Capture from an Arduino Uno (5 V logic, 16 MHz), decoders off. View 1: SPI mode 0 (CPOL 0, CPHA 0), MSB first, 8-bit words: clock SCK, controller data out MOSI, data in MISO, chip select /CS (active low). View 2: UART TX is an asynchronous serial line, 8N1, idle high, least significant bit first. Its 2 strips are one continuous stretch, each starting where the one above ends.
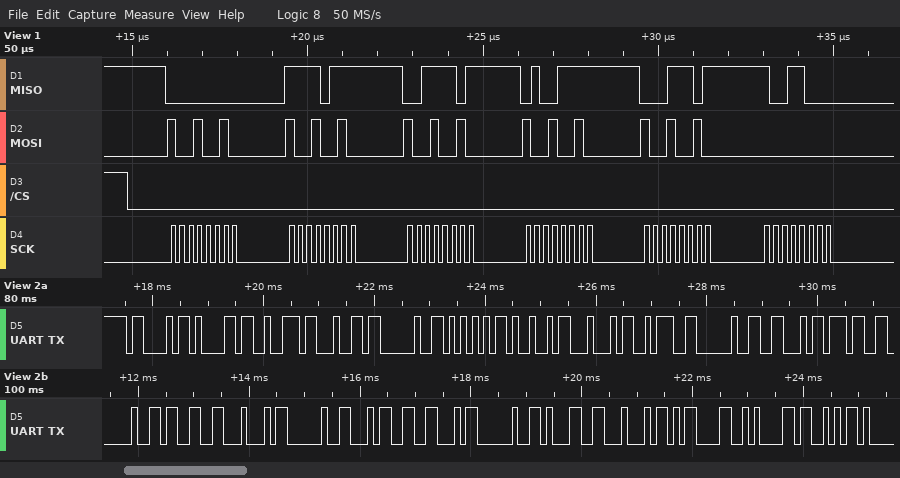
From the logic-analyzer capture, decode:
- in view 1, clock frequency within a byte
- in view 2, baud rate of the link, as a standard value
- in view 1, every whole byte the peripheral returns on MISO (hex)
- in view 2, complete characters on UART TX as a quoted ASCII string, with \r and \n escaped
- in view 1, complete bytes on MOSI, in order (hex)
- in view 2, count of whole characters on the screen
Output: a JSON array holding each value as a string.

["4 MHz", "9600 baud", "00 F7 3D 4F 1D 98", "\"Card UID: F7 3D 4F 1D\\r\\nS\"", "92 92 92 92 92 00", "24"]
